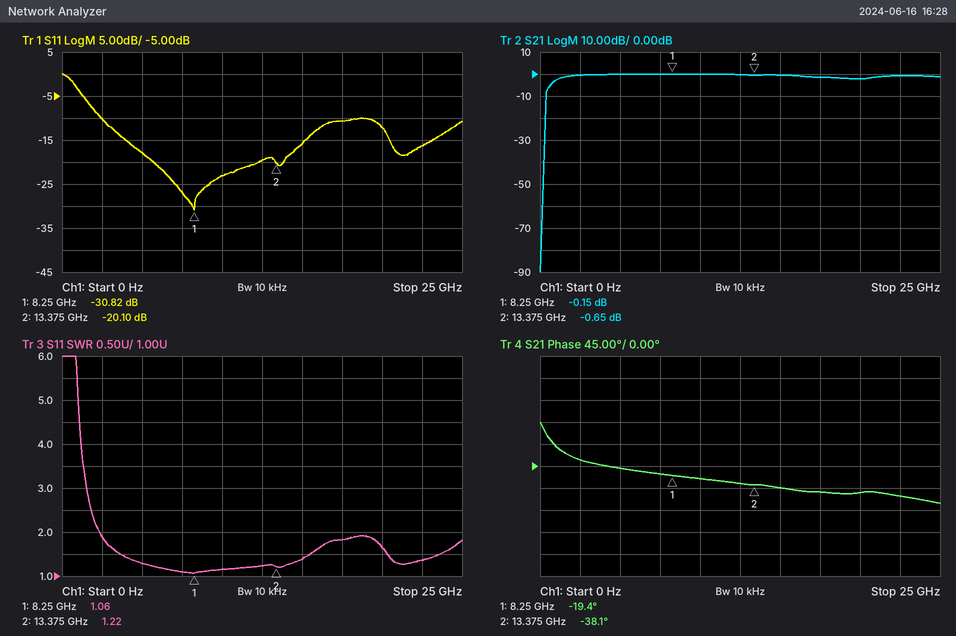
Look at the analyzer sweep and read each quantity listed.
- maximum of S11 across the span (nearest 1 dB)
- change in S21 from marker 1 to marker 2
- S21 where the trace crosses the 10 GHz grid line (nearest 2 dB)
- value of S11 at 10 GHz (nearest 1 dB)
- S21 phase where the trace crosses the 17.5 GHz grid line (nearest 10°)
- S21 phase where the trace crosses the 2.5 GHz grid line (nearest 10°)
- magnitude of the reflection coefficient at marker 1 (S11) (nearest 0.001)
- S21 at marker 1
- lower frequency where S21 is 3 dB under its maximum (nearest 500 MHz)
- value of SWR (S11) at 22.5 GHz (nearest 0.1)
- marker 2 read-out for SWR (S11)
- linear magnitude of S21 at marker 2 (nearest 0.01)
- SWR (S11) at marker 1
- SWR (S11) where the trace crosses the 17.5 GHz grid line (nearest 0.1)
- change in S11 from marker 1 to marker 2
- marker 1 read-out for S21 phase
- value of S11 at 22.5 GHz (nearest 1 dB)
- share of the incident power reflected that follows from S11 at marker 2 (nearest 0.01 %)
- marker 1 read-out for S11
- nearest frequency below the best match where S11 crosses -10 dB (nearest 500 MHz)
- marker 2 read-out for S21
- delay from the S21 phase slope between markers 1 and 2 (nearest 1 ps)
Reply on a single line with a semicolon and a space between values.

0 dB; -0.50 dB; 0 dB; -23 dB; -50°; 10°; 0.029; -0.15 dB; 1.0 GHz; 1.4; 1.22; 0.93; 1.06; 1.8; 10.72 dB; -19.4°; -16 dB; 0.98 %; -30.82 dB; 2.5 GHz; -0.65 dB; 10 ps
